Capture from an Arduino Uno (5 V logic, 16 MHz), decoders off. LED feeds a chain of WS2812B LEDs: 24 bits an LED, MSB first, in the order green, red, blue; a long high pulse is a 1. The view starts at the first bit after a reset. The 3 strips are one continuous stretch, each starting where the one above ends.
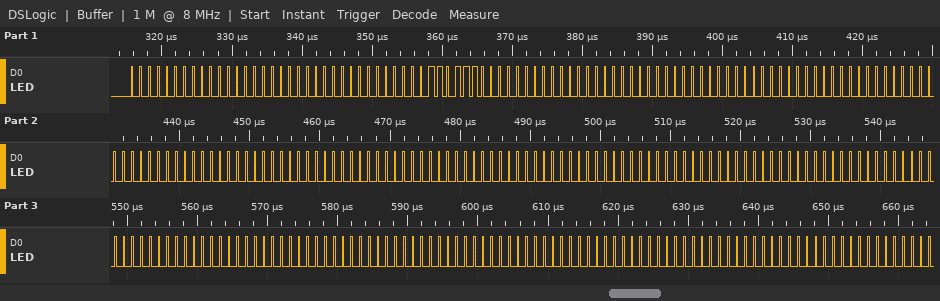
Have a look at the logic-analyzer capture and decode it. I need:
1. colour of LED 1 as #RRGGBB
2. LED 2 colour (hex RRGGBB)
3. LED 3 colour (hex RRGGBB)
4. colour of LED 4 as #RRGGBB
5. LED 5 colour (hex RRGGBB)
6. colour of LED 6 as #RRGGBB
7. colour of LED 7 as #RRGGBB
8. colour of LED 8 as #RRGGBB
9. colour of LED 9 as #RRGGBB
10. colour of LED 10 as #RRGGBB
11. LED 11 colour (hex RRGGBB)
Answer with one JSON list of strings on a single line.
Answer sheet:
["#000000", "#370000", "#000000", "#000000", "#000000", "#000000", "#000000", "#000000", "#000000", "#000000", "#000000"]
